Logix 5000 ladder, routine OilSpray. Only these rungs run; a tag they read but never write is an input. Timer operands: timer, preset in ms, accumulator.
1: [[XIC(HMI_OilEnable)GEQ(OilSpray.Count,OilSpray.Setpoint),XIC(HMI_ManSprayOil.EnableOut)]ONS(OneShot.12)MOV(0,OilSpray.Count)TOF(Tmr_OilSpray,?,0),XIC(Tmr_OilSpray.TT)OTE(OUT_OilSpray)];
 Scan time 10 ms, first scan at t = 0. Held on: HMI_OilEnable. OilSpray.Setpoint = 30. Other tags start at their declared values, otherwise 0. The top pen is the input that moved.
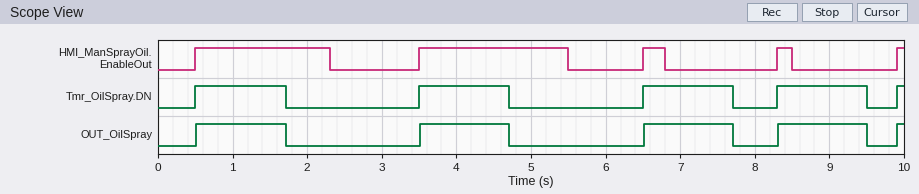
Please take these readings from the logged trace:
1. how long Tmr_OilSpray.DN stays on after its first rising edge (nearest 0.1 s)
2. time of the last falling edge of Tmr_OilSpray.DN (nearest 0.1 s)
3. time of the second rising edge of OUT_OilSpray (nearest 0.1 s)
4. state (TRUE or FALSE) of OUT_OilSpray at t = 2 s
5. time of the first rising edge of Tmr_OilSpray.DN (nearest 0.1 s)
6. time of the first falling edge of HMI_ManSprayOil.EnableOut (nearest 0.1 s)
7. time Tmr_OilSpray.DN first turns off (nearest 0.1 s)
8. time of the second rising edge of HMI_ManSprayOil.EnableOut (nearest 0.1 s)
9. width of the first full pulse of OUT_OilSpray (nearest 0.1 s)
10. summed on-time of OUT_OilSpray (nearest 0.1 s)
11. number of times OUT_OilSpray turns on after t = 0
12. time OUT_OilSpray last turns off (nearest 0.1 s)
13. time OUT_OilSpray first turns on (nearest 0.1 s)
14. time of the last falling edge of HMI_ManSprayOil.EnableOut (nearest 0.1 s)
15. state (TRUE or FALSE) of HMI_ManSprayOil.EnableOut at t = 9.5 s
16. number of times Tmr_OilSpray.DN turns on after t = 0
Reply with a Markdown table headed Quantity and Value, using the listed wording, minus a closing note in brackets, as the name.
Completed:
| Quantity | Value |
|---|---|
| how long Tmr_OilSpray.DN stays on after its first rising edge | 1.2 s |
| time of the last falling edge of Tmr_OilSpray.DN | 9.5 s |
| time of the second rising edge of OUT_OilSpray | 3.5 s |
| state (TRUE or FALSE) of OUT_OilSpray at t = 2 s | FALSE |
| time of the first rising edge of Tmr_OilSpray.DN | 0.5 s |
| time of the first falling edge of HMI_ManSprayOil.EnableOut | 2.3 s |
| time Tmr_OilSpray.DN first turns off | 1.7 s |
| time of the second rising edge of HMI_ManSprayOil.EnableOut | 3.5 s |
| width of the first full pulse of OUT_OilSpray | 1.2 s |
| summed on-time of OUT_OilSpray | 4.9 s |
| number of times OUT_OilSpray turns on after t = 0 | 5 |
| time OUT_OilSpray last turns off | 9.5 s |
| time OUT_OilSpray first turns on | 0.5 s |
| time of the last falling edge of HMI_ManSprayOil.EnableOut | 8.5 s |
| state (TRUE or FALSE) of HMI_ManSprayOil.EnableOut at t = 9.5 s | FALSE |
| number of times Tmr_OilSpray.DN turns on after t = 0 | 5 |
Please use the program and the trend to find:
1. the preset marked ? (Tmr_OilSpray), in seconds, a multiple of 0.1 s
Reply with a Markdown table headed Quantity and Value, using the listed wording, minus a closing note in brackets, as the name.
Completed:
| Quantity | Value |
|---|---|
| the preset marked ? (Tmr_OilSpray), in seconds, a multiple of 0.1 s | 1.2 s |
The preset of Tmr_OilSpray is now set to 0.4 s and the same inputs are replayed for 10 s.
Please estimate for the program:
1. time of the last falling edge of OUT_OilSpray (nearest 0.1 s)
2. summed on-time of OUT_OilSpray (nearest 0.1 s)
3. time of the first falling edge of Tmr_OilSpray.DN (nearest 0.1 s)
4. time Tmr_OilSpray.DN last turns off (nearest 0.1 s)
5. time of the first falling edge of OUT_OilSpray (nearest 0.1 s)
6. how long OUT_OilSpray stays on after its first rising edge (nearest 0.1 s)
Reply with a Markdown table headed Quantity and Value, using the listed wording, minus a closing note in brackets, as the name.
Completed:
| Quantity | Value |
|---|---|
| time of the last falling edge of OUT_OilSpray | 8.7 s |
| summed on-time of OUT_OilSpray | 1.7 s |
| time of the first falling edge of Tmr_OilSpray.DN | 0.9 s |
| time Tmr_OilSpray.DN last turns off | 8.7 s |
| time of the first falling edge of OUT_OilSpray | 0.9 s |
| how long OUT_OilSpray stays on after its first rising edge | 0.4 s |
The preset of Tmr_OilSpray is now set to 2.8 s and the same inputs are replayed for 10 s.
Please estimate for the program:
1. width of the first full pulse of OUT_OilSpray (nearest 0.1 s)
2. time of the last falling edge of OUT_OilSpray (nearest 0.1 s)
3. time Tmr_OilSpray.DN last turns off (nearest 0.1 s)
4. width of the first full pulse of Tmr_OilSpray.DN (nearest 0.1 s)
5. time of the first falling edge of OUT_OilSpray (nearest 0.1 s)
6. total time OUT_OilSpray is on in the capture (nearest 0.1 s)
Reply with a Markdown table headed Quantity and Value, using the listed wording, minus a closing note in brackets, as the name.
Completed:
| Quantity | Value |
|---|---|
| width of the first full pulse of OUT_OilSpray | 2.8 s |
| time of the last falling edge of OUT_OilSpray | 9.9 s |
| time Tmr_OilSpray.DN last turns off | 6.3 s |
| width of the first full pulse of Tmr_OilSpray.DN | 2.8 s |
| time of the first falling edge of OUT_OilSpray | 3.3 s |
| total time OUT_OilSpray is on in the capture | 9.1 s |
